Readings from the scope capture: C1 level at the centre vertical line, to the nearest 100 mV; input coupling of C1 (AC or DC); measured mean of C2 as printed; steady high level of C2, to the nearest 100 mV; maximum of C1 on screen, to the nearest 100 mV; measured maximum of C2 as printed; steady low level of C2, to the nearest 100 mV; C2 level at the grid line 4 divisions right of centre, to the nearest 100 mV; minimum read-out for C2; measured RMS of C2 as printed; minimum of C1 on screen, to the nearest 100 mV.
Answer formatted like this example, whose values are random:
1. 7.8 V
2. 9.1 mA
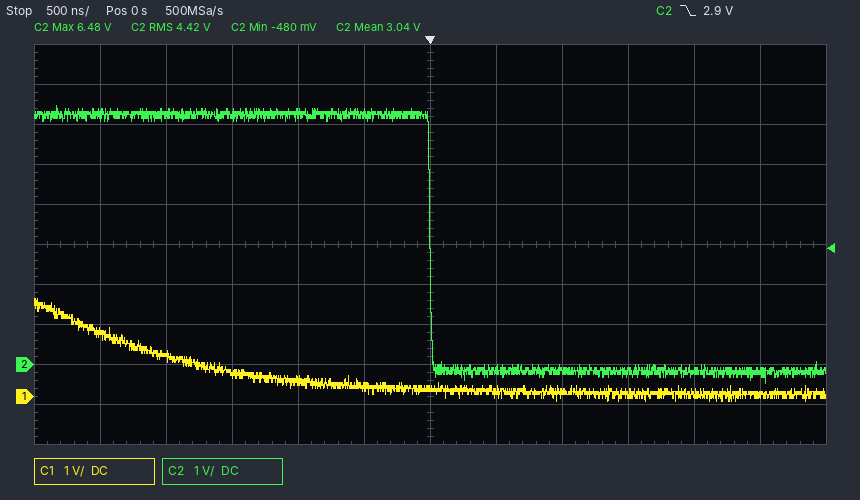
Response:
1. 200 mV
2. DC
3. 3.04 V
4. 6.2 V
5. 2.4 V
6. 6.48 V
7. -200 mV
8. -200 mV
9. -480 mV
10. 4.42 V
11. -100 mV
